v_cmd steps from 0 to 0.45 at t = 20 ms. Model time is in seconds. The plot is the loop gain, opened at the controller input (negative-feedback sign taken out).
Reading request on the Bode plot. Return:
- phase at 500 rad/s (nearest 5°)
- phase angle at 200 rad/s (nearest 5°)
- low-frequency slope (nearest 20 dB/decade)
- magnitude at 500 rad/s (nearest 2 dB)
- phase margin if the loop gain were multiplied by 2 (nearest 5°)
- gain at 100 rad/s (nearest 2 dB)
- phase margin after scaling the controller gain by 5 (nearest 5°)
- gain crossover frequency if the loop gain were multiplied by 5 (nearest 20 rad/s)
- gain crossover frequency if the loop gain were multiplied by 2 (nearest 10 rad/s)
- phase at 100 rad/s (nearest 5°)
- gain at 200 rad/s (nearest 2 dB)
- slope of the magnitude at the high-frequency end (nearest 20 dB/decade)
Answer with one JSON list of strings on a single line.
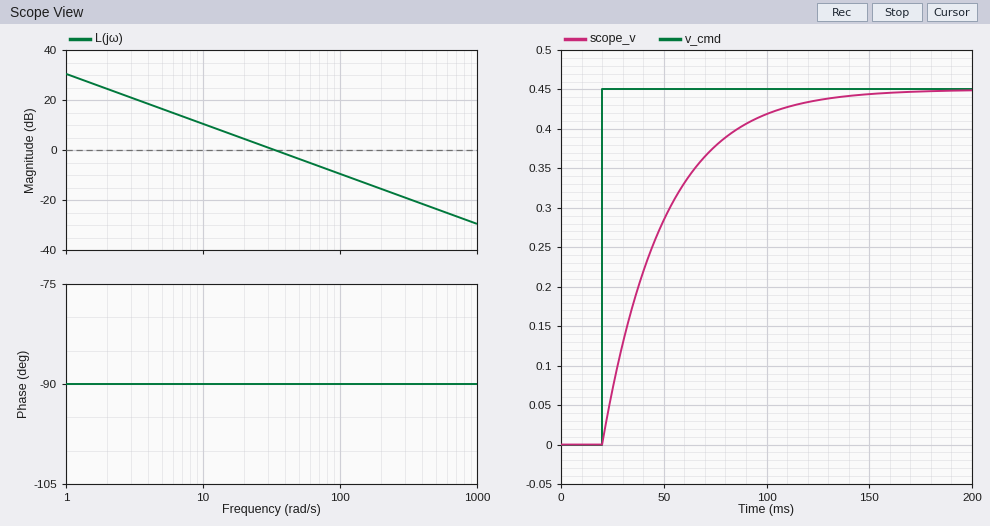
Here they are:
["-90°", "-90°", "-20 dB/decade", "-24 dB", "90°", "-10 dB", "90°", "160 rad/s", "70 rad/s", "-90°", "-16 dB", "-20 dB/decade"]
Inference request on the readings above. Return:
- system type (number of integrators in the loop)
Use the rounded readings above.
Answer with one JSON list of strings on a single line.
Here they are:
["1"]
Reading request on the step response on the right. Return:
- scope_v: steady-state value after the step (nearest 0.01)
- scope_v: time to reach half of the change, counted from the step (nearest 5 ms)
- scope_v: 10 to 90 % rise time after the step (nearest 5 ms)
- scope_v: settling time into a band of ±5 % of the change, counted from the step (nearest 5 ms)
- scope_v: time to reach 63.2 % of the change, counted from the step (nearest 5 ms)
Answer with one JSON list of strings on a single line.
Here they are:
["0.45", "20 ms", "65 ms", "90 ms", "30 ms"]
